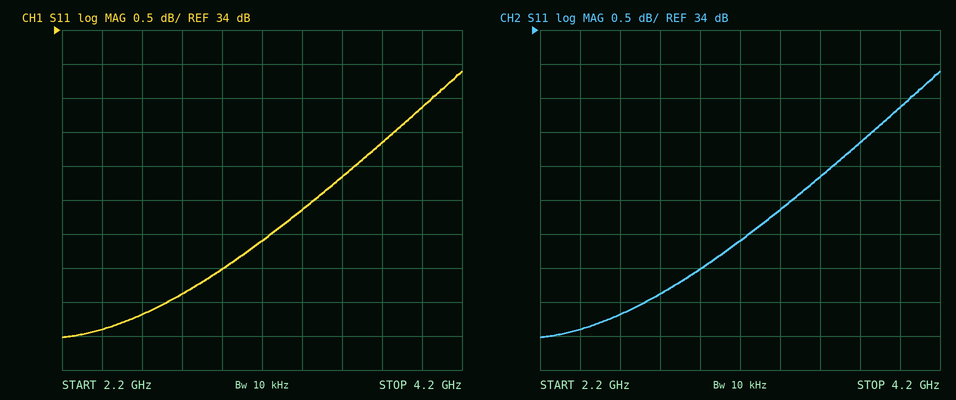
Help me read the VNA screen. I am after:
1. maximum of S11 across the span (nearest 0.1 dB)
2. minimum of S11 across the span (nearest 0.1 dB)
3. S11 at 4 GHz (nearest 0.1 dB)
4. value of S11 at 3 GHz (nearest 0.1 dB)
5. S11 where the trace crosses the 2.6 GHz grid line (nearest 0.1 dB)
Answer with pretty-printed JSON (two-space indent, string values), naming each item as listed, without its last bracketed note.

{
  "maximum of S11 across the span": "33.4 dB",
  "minimum of S11 across the span": "29.5 dB",
  "S11 at 4 GHz": "32.9 dB",
  "value of S11 at 3 GHz": "30.5 dB",
  "S11 where the trace crosses the 2.6 GHz grid line": "29.8 dB"
}
